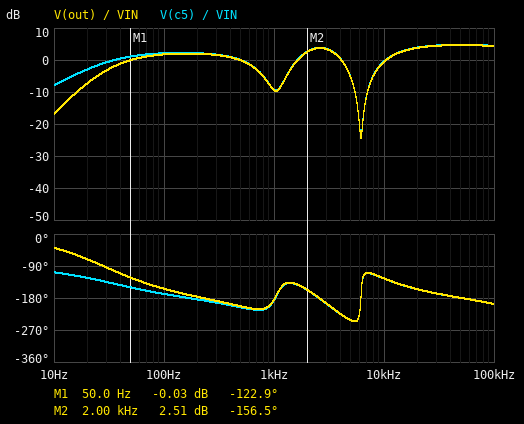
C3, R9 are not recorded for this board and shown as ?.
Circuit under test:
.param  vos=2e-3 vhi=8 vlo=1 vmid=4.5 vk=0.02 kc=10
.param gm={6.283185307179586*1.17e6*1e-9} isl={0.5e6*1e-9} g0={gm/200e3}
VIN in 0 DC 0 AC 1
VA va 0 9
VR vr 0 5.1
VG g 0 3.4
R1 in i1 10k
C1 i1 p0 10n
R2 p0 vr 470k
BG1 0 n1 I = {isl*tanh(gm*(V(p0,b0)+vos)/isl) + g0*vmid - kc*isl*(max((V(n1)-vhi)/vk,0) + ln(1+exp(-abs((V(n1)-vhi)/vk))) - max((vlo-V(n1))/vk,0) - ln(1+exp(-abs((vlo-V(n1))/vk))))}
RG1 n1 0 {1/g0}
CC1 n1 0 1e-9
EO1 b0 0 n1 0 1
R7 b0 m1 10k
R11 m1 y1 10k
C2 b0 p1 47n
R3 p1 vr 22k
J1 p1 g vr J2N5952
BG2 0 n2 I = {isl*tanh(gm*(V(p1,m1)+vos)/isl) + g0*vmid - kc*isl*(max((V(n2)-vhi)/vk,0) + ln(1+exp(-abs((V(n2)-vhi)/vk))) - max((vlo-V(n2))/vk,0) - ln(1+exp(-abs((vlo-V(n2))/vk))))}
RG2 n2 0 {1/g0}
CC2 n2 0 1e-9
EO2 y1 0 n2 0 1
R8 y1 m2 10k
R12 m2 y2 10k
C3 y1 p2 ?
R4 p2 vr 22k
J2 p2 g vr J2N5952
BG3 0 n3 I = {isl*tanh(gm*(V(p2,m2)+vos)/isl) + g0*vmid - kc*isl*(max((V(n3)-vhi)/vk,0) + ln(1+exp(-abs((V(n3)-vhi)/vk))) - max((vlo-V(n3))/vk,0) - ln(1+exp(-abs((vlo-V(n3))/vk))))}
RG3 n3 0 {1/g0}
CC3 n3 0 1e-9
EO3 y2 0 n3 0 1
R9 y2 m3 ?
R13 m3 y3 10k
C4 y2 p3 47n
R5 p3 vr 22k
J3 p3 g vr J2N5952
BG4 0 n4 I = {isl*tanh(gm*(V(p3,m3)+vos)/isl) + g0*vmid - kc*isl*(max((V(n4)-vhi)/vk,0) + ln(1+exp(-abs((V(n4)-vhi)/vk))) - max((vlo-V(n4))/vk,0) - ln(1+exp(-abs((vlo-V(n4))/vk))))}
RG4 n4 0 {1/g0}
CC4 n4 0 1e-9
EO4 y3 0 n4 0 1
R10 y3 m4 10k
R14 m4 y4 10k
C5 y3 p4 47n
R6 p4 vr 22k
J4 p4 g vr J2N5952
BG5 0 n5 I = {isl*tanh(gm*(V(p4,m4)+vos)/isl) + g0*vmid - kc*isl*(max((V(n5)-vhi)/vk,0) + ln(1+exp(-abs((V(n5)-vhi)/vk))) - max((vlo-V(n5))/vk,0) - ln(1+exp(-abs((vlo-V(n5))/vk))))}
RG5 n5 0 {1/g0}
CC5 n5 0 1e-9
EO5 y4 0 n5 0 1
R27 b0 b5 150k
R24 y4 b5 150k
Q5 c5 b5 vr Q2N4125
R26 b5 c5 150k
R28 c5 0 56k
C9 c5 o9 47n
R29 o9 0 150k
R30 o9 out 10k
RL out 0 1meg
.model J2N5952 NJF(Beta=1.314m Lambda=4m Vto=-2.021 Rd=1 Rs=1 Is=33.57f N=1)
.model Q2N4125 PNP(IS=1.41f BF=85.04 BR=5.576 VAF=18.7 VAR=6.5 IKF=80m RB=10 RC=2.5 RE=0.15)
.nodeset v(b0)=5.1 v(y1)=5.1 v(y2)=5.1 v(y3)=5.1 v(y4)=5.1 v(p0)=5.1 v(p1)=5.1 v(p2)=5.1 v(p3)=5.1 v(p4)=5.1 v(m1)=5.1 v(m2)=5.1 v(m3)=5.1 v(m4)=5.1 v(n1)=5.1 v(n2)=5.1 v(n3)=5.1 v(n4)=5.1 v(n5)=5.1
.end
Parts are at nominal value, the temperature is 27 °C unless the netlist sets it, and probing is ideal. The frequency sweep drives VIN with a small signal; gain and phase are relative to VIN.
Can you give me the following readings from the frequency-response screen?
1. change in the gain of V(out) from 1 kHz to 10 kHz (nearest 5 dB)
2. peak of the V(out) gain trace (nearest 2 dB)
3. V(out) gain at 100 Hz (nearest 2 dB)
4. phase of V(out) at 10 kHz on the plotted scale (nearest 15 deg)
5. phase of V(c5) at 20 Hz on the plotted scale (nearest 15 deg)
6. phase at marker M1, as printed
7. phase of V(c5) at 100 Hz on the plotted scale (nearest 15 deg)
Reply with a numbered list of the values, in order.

1. 10 dB
2. 4 dB
3. 2 dB
4. -120 deg
5. -120 deg
6. -122.9 deg
7. -165 deg
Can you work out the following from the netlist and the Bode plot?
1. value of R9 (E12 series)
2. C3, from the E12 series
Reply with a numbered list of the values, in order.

1. 18 kΩ
2. 68 nF
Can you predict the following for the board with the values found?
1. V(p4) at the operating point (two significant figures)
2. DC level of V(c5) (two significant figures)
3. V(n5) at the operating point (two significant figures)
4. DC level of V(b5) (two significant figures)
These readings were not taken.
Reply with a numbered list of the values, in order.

1. 5.1 V
2. 3.1 V
3. 5.1 V
4. 4.5 V
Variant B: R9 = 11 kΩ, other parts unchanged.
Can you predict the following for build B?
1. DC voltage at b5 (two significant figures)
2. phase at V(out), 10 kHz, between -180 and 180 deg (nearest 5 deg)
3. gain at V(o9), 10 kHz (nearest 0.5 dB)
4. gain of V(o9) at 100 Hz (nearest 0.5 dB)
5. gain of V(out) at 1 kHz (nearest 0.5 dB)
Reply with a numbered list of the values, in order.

1. 4.5 V
2. -120 deg
3. -1.0 dB
4. 3.5 dB
5. -12.5 dB
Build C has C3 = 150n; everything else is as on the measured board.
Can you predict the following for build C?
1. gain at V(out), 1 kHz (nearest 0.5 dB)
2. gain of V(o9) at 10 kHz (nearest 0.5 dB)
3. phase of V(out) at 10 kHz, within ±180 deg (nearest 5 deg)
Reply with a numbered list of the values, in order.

1. -5.5 dB
2. 1.0 dB
3. -130 deg
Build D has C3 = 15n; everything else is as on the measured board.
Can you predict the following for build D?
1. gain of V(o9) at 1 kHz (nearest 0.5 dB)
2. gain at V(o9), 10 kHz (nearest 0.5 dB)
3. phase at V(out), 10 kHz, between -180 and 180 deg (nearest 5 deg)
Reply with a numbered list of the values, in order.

1. -4.0 dB
2. -23.5 dB
3. -115 deg
